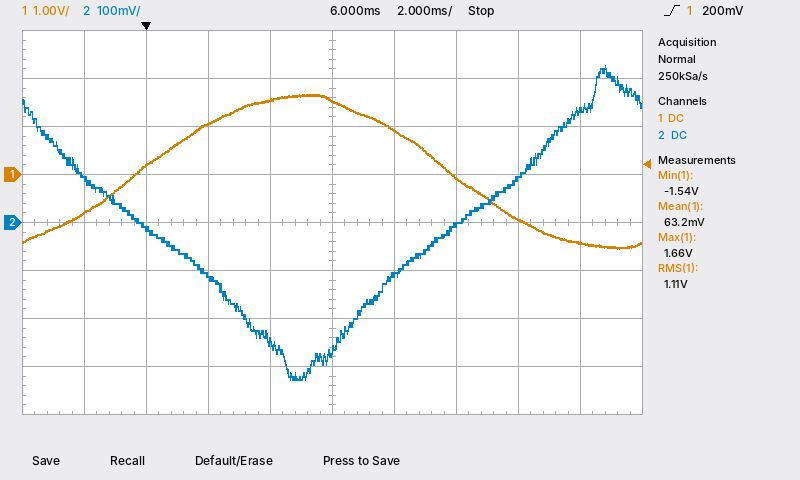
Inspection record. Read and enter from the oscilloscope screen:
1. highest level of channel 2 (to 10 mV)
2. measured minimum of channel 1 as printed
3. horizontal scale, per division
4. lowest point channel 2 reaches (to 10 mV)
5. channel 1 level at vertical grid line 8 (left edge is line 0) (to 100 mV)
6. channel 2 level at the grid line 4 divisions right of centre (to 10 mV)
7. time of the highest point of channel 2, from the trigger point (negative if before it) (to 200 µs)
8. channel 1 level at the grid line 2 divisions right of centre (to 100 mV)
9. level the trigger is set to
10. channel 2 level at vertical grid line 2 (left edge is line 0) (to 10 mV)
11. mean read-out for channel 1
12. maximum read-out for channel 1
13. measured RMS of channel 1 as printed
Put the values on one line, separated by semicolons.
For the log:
330 mV; -1.54 V; 2 ms; -330 mV; -900 mV; 230 mV; +14.8 ms; -100 mV; 200 mV; -10 mV; 63.2 mV; 1.66 V; 1.11 V
